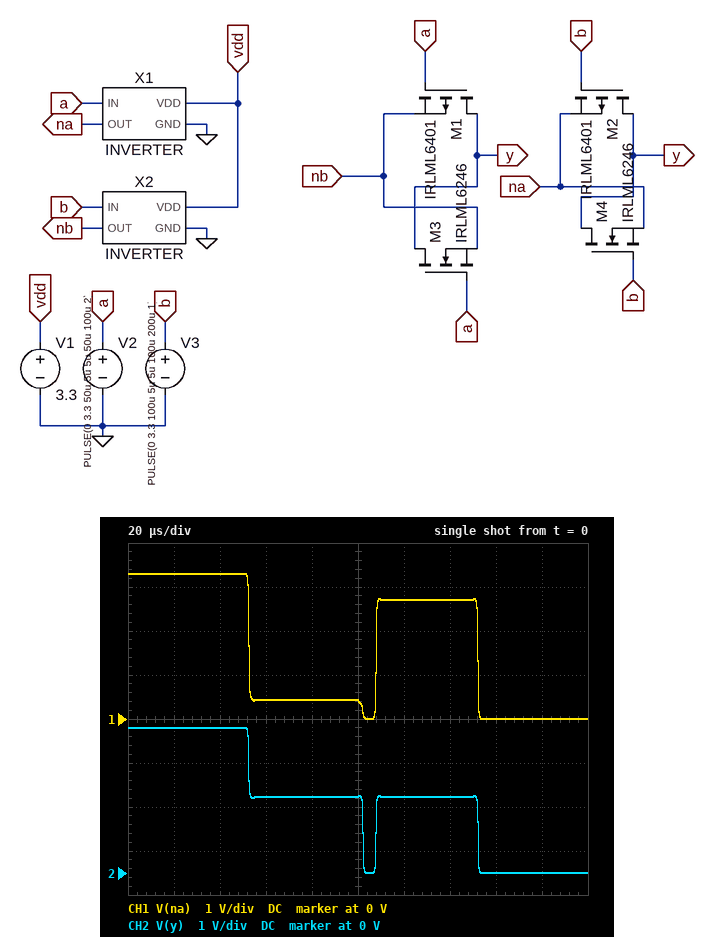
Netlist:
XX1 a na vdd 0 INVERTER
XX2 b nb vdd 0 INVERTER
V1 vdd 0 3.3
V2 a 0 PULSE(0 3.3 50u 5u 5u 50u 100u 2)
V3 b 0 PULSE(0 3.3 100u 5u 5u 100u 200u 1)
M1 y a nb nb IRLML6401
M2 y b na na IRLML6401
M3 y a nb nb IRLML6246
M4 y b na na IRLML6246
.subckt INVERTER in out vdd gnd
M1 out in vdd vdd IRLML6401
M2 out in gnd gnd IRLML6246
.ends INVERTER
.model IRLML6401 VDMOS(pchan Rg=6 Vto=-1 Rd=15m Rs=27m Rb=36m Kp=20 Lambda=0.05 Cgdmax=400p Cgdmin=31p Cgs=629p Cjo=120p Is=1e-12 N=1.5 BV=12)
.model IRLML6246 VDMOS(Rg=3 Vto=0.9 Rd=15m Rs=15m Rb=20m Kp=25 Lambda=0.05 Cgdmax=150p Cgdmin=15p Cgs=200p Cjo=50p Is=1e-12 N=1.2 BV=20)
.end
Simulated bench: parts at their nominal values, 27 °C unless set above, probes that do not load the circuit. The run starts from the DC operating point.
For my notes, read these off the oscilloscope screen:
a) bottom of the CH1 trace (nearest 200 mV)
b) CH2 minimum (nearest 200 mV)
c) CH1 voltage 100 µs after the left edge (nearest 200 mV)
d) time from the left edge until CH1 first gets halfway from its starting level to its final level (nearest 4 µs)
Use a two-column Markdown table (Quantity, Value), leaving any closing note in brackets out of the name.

| Quantity | Value |
|---|---|
| bottom of the CH1 trace | 0 V |
| CH2 minimum | 0 V |
| CH1 voltage 100 µs after the left edge | 400 mV |
| time from the left edge until CH1 first gets halfway from its starting level to its final level | 52 µs |
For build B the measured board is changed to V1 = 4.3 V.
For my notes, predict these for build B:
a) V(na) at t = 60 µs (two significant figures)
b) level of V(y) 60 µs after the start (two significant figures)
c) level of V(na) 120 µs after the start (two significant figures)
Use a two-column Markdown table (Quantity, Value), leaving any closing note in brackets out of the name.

| Quantity | Value |
|---|---|
| V(na) at t = 60 µs | 770 mV |
| level of V(y) 60 µs after the start | 2.1 V |
| level of V(na) 120 µs after the start | 3.4 V |
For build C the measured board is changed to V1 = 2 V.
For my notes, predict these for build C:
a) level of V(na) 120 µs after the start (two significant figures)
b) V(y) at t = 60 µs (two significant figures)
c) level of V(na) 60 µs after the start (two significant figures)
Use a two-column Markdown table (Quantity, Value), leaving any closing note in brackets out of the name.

| Quantity | Value |
|---|---|
| level of V(na) 120 µs after the start | 1.6 V |
| V(y) at t = 60 µs | 1.4 V |
| level of V(na) 60 µs after the start | 170 mV |
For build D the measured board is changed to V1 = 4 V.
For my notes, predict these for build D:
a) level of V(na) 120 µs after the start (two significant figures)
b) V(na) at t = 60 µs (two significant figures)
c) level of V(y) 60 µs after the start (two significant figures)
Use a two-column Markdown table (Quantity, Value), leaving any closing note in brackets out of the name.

| Quantity | Value |
|---|---|
| level of V(na) 120 µs after the start | 3.2 V |
| V(na) at t = 60 µs | 660 mV |
| level of V(y) 60 µs after the start | 2.0 V |
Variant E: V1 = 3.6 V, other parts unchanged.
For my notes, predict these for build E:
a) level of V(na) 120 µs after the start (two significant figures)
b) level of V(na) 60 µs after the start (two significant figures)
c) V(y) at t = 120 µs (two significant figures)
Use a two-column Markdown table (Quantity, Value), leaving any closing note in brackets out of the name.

| Quantity | Value |
|---|---|
| level of V(na) 120 µs after the start | 2.9 V |
| level of V(na) 60 µs after the start | 520 mV |
| V(y) at t = 120 µs | 1.8 V |
